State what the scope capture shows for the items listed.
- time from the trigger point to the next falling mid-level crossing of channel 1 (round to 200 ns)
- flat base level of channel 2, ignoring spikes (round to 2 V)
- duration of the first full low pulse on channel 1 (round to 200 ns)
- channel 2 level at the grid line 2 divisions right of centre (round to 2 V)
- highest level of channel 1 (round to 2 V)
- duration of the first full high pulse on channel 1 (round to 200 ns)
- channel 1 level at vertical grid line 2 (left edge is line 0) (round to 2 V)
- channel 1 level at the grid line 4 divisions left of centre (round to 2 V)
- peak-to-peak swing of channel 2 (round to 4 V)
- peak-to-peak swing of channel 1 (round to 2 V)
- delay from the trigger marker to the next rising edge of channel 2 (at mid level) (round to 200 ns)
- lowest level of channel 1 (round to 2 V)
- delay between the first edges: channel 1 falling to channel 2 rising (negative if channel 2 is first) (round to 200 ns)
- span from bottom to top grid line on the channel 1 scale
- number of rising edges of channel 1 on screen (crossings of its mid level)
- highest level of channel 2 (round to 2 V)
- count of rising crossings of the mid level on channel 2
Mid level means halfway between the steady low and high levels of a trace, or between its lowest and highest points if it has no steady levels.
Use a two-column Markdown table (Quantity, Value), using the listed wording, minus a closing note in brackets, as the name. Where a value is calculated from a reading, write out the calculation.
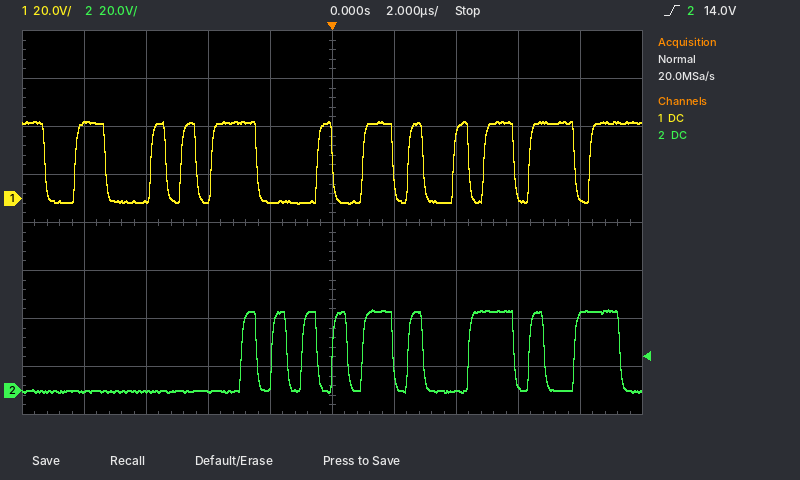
| Quantity | Value |
|---|---|
| time from the trigger point to the next falling mid-level crossing of channel 1 | 2.0 µs |
| flat base level of channel 2, ignoring spikes | 0 V |
| duration of the first full low pulse on channel 1 | 1.0 µs |
| channel 2 level at the grid line 2 divisions right of centre | 0 V |
| highest level of channel 1 | 32 V |
| duration of the first full high pulse on channel 1 | 1.0 µs |
| channel 1 level at vertical grid line 2 (left edge is line 0) | 0 V |
| channel 1 level at the grid line 4 divisions left of centre | 32 V |
| peak-to-peak swing of channel 2 | 36 V |
| peak-to-peak swing of channel 1 | 32 V − (-2 V) = 34 V |
| delay from the trigger marker to the next rising edge of channel 2 (at mid level) | 1.0 µs |
| lowest level of channel 1 | -2 V |
| delay between the first edges: channel 1 falling to channel 2 rising (negative if channel 2 is first) | +6.4 µs |
| span from bottom to top grid line on the channel 1 scale | 160 V |
| number of rising edges of channel 1 on screen | 11 |
| highest level of channel 2 | 34 V |
| count of rising crossings of the mid level on channel 2 | 9 |
